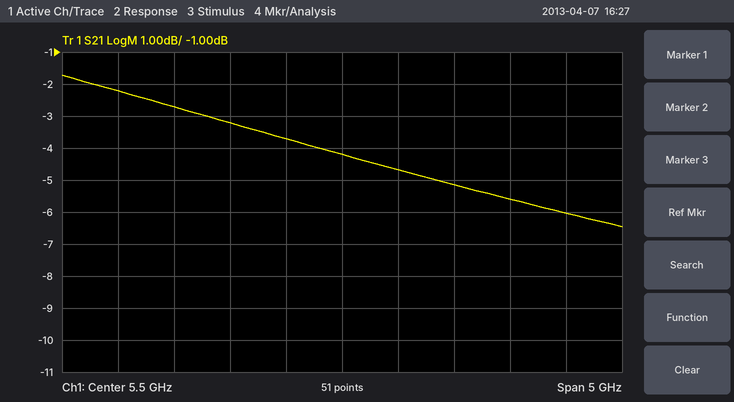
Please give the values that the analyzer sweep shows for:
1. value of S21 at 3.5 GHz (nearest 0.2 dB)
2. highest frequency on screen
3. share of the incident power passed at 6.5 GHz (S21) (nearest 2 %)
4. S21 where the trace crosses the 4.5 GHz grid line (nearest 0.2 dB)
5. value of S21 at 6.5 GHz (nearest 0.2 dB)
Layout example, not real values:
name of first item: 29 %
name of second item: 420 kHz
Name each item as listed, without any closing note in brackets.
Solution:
value of S21 at 3.5 GHz: -2.2 dB
highest frequency on screen: 8 GHz
share of the incident power passed at 6.5 GHz (S21): 30 %
S21 where the trace crosses the 4.5 GHz grid line: -3.2 dB
value of S21 at 6.5 GHz: -5.2 dB
